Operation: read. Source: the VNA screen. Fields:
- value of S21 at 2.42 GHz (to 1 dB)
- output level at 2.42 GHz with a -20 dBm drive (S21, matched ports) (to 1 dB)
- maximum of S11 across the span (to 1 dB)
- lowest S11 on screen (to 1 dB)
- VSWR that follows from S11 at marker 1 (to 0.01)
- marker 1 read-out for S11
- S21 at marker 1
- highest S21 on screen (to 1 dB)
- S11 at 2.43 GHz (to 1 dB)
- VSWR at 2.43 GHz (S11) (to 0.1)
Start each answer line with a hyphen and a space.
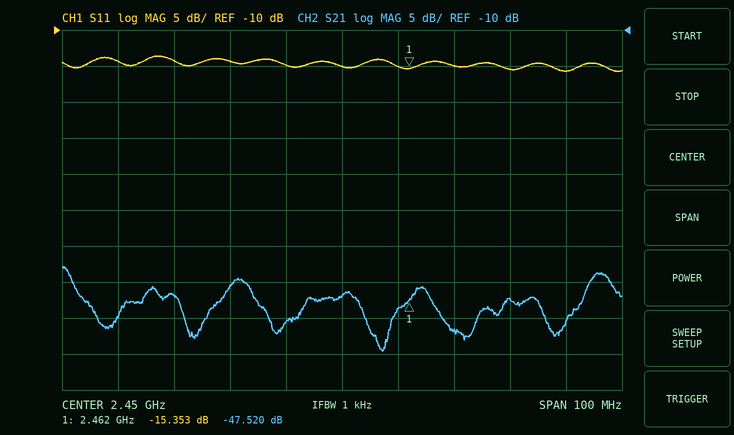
- -47 dB
- -67 dBm
- -14 dB
- -16 dB
- 1.41
- -15.353 dB
- -47.520 dB
- -43 dB
- -14 dB
- 1.5
